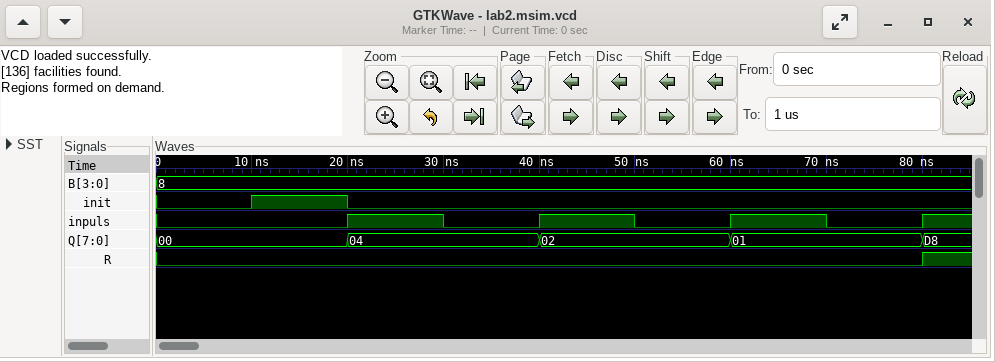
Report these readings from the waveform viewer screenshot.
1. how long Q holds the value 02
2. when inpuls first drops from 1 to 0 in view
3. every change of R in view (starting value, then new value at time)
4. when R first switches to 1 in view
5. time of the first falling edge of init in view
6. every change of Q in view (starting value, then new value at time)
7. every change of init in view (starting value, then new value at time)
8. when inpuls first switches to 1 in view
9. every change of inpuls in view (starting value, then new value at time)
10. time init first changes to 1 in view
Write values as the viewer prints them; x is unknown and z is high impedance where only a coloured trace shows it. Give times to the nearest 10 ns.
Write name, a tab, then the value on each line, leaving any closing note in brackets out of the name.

how long Q holds the value 02	20 ns
when inpuls first drops from 1 to 0 in view	30 ns
every change of R in view	0, 1 at 80 ns
when R first switches to 1 in view	80 ns
time of the first falling edge of init in view	20 ns
every change of Q in view	00, 04 at 20 ns, 02 at 40 ns, 01 at 60 ns, D8 at 80 ns
every change of init in view	0, 1 at 10 ns, 0 at 20 ns
when inpuls first switches to 1 in view	20 ns
every change of inpuls in view	0, 1 at 20 ns, 0 at 30 ns, 1 at 40 ns, 0 at 50 ns, 1 at 60 ns, 0 at 70 ns, 1 at 80 ns
time init first changes to 1 in view	10 ns
